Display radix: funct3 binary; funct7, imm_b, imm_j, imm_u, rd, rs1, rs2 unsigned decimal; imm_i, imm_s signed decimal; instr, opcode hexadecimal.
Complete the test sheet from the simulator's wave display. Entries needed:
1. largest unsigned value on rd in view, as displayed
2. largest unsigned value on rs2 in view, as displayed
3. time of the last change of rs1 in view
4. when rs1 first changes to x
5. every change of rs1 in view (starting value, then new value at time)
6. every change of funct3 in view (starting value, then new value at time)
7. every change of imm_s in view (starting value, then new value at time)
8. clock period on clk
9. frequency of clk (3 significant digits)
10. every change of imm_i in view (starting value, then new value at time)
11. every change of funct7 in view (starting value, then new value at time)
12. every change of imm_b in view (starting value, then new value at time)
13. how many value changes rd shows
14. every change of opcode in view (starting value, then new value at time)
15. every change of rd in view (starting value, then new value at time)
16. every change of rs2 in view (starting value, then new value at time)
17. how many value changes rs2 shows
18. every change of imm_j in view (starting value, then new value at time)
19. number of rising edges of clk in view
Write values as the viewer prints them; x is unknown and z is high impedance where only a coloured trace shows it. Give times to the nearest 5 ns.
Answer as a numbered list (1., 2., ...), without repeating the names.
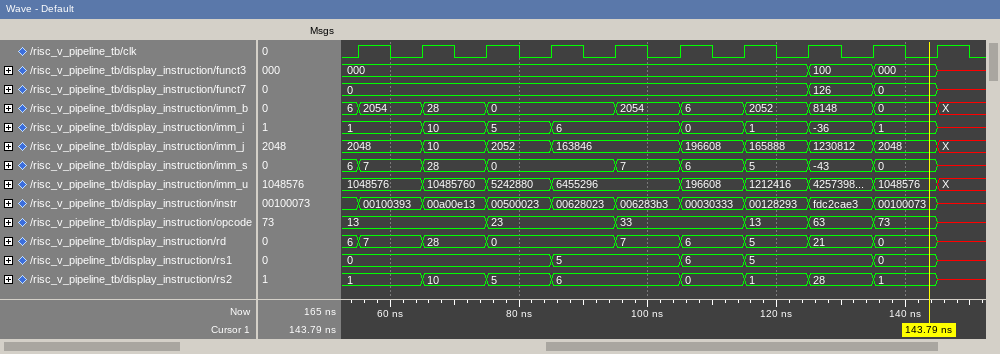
1. 28
2. 28
3. 145 ns
4. 145 ns
5. 0, 5 at 85 ns, 6 at 105 ns, 5 at 115 ns, 0 at 135 ns, x at 145 ns
6. 000, 100 at 125 ns, 000 at 135 ns, x at 145 ns
7. 6, 7 at 55 ns, 28 at 65 ns, 0 at 75 ns, 7 at 95 ns, 6 at 105 ns, 5 at 115 ns, -43 at 125 ns, 0 at 135 ns, x at 145 ns
8. 10 ns
9. 100 MHz
10. 1, 10 at 65 ns, 5 at 75 ns, 6 at 85 ns, 0 at 105 ns, 1 at 115 ns, -36 at 125 ns, 1 at 135 ns, x at 145 ns
11. 0, 126 at 125 ns, 0 at 135 ns, x at 145 ns
12. 6, 2054 at 55 ns, 28 at 65 ns, 0 at 75 ns, 2054 at 95 ns, 6 at 105 ns, 2052 at 115 ns, 8148 at 125 ns, 0 at 135 ns, X at 145 ns
13. 9
14. 13, 23 at 75 ns, 33 at 95 ns, 13 at 115 ns, 63 at 125 ns, 73 at 135 ns, x at 145 ns
15. 6, 7 at 55 ns, 28 at 65 ns, 0 at 75 ns, 7 at 95 ns, 6 at 105 ns, 5 at 115 ns, 21 at 125 ns, 0 at 135 ns, x at 145 ns
16. 1, 10 at 65 ns, 5 at 75 ns, 6 at 85 ns, 0 at 105 ns, 1 at 115 ns, 28 at 125 ns, 1 at 135 ns, x at 145 ns
17. 8
18. 2048, 10 at 65 ns, 2052 at 75 ns, 163846 at 85 ns, 196608 at 105 ns, 165888 at 115 ns, 1230812 at 125 ns, 2048 at 135 ns, X at 145 ns
19. 10
